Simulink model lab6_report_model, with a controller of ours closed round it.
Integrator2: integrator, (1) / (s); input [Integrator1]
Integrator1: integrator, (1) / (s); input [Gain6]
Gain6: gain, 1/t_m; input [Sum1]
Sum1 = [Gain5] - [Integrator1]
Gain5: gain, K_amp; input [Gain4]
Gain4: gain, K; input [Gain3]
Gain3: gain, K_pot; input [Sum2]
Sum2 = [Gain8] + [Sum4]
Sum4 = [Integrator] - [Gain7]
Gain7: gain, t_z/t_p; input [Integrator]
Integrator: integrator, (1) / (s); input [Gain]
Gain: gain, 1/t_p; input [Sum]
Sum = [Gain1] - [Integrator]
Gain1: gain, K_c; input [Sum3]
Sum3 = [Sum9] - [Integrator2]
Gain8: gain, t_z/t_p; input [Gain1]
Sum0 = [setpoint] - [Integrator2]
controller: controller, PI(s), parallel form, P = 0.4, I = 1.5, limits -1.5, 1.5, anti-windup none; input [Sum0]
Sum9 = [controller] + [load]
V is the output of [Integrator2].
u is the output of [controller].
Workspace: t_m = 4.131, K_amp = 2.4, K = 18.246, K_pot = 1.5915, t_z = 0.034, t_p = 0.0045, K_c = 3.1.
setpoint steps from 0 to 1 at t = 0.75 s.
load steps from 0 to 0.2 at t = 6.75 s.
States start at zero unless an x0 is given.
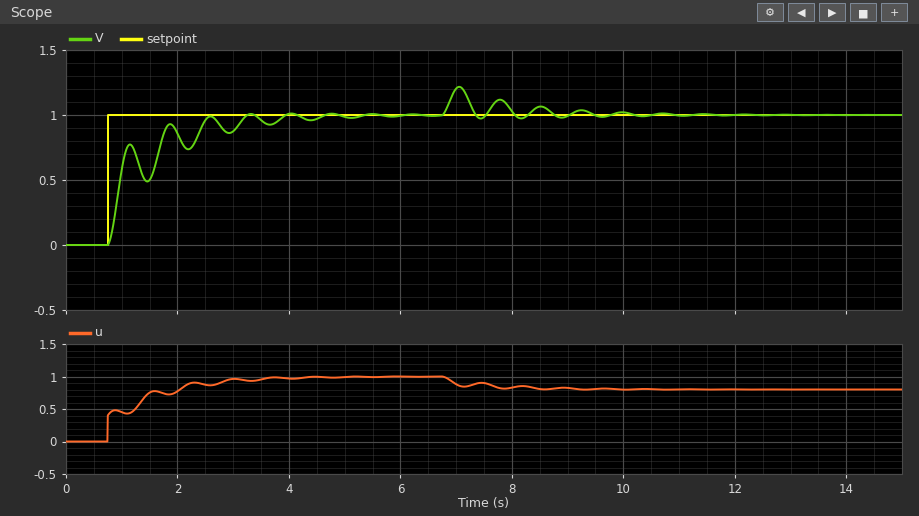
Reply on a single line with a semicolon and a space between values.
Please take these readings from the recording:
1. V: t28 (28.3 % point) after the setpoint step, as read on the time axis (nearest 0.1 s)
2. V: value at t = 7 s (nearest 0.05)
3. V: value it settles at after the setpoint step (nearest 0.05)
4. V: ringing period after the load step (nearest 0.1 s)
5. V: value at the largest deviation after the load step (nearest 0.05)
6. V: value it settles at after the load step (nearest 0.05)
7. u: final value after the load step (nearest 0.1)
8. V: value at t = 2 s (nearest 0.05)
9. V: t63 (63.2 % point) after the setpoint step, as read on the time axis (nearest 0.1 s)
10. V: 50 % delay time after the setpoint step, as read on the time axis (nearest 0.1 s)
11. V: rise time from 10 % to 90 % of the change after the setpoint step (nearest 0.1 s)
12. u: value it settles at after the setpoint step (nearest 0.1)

0.9 s; 1.20; 1.00; 0.7 s; 1.20; 1.00; 0.8; 0.85; 1.0 s; 1.0 s; 1.0 s; 1.0
